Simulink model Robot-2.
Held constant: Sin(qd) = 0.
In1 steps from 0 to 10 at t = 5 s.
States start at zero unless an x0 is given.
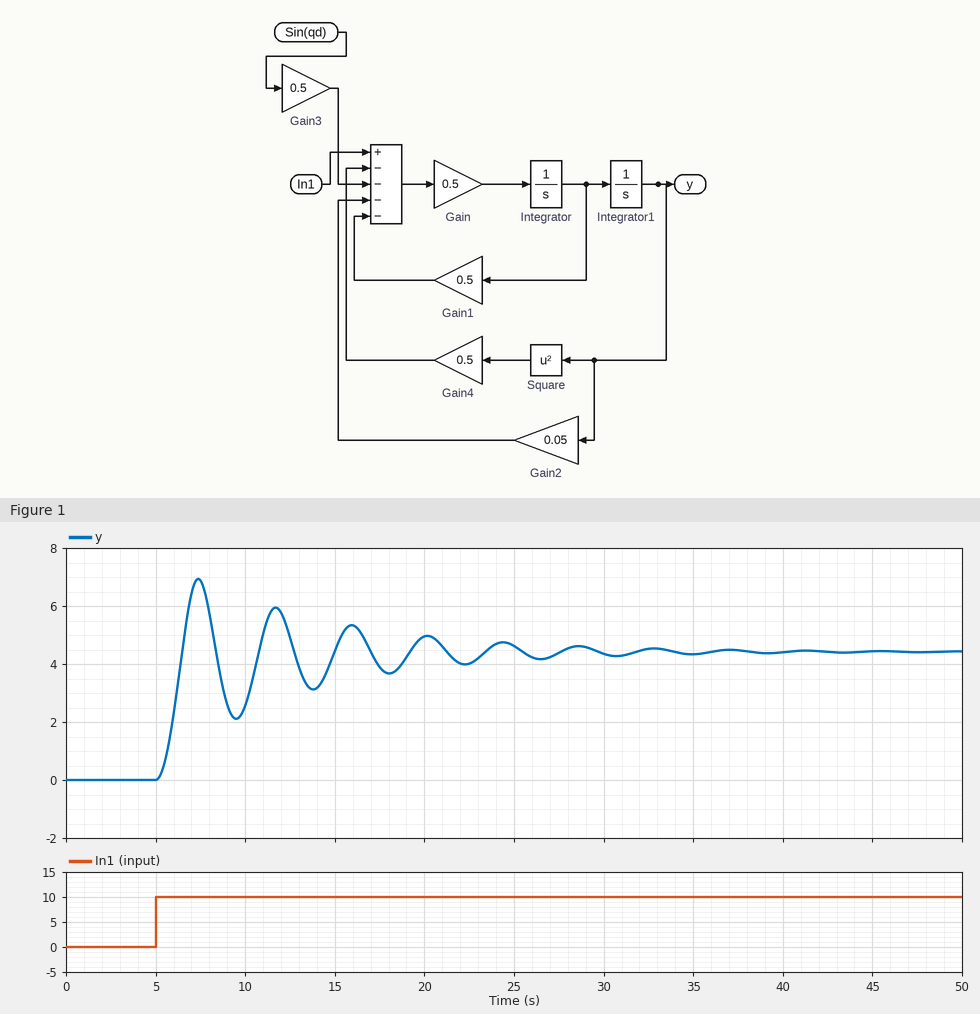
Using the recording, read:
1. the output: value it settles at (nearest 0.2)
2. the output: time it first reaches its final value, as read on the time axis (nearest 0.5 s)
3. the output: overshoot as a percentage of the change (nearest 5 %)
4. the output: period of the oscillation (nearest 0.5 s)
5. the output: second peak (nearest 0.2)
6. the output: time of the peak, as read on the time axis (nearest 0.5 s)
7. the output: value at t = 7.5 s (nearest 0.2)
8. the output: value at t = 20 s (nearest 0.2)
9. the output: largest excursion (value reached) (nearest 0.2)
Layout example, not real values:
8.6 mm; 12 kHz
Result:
4.4; 6.5 s; 55 %; 4.5 s; 6.0; 7.5 s; 6.8; 5.0; 7.0
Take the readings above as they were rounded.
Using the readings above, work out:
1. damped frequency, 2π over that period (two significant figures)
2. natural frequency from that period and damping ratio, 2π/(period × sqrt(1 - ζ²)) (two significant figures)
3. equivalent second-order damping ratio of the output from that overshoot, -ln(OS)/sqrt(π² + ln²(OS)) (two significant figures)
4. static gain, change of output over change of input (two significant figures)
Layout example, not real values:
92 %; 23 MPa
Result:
1.4 rad/s; 1.4 rad/s; 0.19; 0.44
